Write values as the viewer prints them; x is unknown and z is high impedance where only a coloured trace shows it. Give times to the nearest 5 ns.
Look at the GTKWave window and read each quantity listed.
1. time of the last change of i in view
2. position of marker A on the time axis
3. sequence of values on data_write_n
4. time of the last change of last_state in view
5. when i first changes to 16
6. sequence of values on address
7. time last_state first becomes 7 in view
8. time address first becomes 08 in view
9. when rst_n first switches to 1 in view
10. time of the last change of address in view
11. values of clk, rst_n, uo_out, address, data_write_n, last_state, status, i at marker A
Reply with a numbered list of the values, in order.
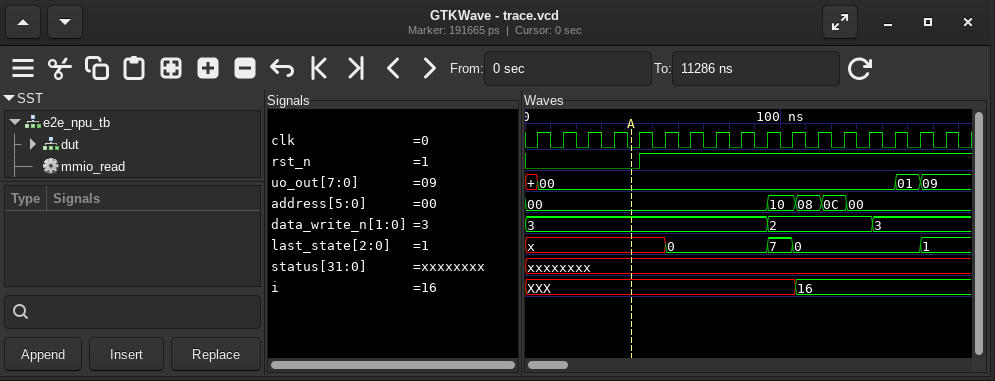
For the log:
1. 105 ns
2. 40 ns
3. 3, 2, 3
4. 155 ns
5. 105 ns
6. 00, 10, 08, 0C, 00
7. 95 ns
8. 105 ns
9. 45 ns
10. 125 ns
11. clk=0, rst_n=0, uo_out=00, address=00, data_write_n=3, last_state=x, status=xxxxxxxx, i=XXX
